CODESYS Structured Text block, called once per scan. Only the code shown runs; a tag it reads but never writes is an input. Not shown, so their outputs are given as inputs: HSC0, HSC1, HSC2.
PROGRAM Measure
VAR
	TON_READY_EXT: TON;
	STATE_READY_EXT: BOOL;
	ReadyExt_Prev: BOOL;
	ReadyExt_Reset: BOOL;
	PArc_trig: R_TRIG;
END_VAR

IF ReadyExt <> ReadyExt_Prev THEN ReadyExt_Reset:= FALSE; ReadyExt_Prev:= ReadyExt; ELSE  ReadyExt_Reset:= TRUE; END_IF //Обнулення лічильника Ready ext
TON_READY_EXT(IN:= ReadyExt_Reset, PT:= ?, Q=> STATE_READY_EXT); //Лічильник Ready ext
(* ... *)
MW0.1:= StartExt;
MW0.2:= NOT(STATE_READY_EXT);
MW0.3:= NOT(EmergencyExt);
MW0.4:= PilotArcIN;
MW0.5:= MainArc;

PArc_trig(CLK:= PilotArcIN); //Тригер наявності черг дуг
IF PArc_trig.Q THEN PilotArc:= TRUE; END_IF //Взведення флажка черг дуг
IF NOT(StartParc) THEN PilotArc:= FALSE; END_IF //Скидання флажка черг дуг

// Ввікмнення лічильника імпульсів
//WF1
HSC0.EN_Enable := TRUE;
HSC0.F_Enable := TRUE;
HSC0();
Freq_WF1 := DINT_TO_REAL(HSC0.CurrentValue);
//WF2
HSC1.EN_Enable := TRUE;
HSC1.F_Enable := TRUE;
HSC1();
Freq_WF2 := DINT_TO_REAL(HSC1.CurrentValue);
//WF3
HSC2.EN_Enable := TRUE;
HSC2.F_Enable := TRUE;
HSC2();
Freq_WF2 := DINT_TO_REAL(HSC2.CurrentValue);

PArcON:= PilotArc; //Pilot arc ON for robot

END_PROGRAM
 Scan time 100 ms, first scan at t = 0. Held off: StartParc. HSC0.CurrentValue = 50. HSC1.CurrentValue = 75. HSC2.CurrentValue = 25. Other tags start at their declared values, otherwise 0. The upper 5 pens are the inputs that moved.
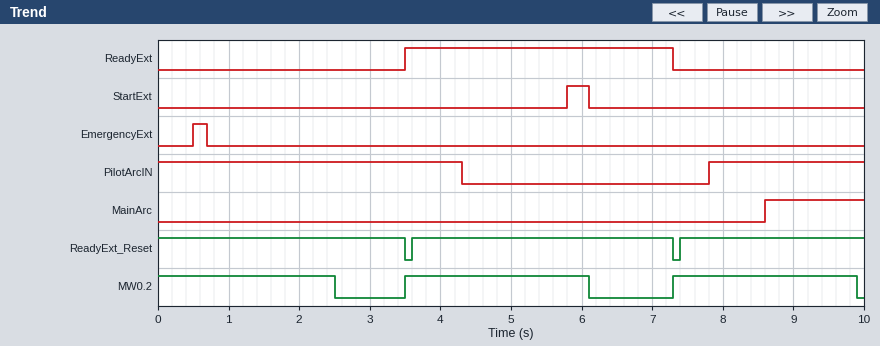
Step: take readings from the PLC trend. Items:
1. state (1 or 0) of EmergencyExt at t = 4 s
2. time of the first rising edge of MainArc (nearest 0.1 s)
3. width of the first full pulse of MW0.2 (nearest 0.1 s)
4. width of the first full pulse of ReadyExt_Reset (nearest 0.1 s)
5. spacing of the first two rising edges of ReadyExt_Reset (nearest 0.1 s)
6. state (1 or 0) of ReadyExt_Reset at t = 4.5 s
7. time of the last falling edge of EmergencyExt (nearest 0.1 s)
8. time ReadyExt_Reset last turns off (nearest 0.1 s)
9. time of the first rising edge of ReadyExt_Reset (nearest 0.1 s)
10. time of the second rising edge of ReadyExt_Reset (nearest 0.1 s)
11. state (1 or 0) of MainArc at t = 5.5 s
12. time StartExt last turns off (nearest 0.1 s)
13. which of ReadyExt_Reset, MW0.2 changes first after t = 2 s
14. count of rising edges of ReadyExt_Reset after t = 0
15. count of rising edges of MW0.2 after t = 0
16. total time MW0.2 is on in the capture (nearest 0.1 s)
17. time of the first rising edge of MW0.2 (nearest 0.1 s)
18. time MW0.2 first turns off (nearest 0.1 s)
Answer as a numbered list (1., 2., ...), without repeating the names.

1. 0
2. 8.6 s
3. 2.6 s
4. 3.7 s
5. 3.8 s
6. 1
7. 0.7 s
8. 7.3 s
9. 3.6 s
10. 7.4 s
11. 0
12. 6.1 s
13. MW0.2
14. 2
15. 2
16. 7.7 s
17. 3.5 s
18. 2.5 s
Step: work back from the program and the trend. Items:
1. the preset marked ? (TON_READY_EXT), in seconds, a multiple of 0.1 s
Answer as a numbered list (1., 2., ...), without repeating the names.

1. 2.5 s
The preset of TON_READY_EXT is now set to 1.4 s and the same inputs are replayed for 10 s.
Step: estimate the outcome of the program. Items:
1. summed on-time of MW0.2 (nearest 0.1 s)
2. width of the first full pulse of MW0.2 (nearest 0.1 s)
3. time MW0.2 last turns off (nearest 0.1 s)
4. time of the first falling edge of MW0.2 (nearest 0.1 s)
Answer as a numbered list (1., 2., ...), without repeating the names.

1. 4.4 s
2. 1.5 s
3. 8.8 s
4. 1.4 s
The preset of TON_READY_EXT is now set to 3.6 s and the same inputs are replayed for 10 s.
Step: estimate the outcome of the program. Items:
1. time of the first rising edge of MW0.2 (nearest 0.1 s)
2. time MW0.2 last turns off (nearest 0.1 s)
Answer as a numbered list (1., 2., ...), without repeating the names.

1. 7.3 s
2. 7.2 s
